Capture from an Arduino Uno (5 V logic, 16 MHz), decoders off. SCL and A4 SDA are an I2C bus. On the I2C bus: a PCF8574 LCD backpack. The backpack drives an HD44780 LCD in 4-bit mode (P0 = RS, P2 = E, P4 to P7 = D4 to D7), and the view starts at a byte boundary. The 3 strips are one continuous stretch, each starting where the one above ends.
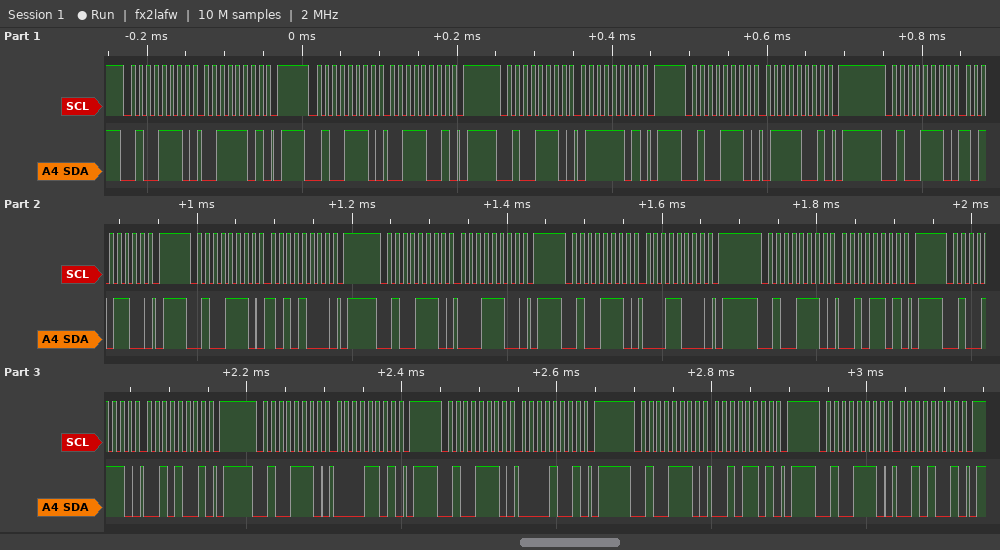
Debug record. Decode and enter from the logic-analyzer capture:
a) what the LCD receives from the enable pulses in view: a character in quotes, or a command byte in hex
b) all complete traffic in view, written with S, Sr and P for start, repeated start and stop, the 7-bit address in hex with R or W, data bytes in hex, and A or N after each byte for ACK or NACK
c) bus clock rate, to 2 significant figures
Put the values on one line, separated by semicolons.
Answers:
'7' 0xA1 ' '; S 27W A 3D A P S 27W A 39 A P S 27W A 7D A P S 27W A 79 A P S 27W A AC A P S 27W A A8 A P S 27W A 1C A P S 27W A 18 A P S 27W A 2D A P S 27W A 29 A P S 27W A 0D A P S 27W A 09 A P S 27W A 2D A P S 27W A 29 A P; 100 kHz
